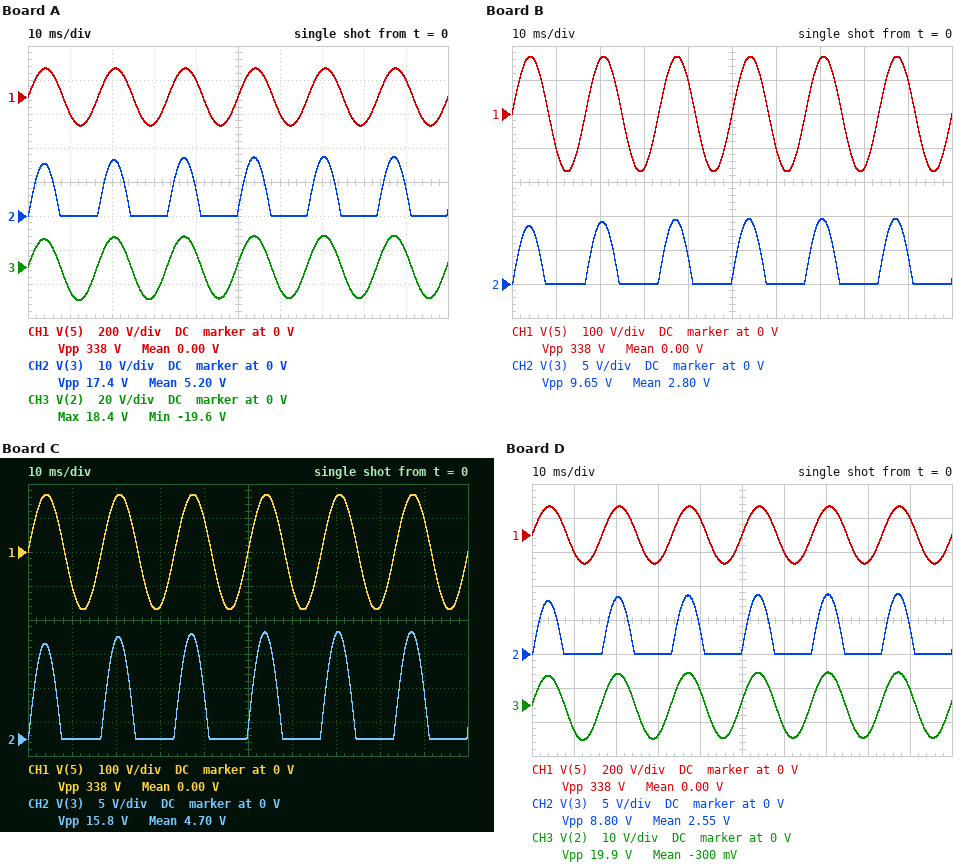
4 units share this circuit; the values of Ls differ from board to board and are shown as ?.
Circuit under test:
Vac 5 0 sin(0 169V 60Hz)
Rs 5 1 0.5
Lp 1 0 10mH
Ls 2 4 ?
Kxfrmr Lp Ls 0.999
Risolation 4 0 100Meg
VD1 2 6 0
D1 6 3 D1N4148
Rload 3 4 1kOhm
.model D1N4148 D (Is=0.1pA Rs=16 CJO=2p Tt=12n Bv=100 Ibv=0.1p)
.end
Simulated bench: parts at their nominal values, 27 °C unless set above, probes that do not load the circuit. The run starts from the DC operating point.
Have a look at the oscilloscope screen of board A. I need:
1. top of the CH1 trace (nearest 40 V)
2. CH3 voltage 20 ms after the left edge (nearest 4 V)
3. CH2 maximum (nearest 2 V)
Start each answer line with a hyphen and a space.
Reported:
- 160 V
- 16 V
- 18 V
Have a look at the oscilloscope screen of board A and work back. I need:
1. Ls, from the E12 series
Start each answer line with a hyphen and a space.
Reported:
- 120 µH
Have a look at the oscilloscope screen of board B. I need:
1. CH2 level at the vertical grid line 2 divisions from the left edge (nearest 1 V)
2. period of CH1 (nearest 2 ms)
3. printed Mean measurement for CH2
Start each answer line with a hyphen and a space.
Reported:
- 9 V
- 16 ms
- 2.80 V
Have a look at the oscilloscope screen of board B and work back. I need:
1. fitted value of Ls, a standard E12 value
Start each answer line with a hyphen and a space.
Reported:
- 39 µH
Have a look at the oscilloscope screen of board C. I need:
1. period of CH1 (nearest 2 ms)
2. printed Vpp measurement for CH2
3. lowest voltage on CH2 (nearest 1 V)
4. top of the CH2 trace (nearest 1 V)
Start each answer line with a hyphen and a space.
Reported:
- 16 ms
- 15.8 V
- 0 V
- 16 V
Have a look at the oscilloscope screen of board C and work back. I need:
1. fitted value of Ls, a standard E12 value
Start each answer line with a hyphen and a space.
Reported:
- 100 µH
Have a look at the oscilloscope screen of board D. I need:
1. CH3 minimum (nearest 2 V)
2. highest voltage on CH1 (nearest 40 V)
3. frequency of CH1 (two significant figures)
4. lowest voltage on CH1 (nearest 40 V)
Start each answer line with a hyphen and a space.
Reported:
- -10 V
- 160 V
- 60 Hz
- -160 V
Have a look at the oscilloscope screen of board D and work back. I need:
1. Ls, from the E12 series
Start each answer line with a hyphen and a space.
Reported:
- 33 µH
